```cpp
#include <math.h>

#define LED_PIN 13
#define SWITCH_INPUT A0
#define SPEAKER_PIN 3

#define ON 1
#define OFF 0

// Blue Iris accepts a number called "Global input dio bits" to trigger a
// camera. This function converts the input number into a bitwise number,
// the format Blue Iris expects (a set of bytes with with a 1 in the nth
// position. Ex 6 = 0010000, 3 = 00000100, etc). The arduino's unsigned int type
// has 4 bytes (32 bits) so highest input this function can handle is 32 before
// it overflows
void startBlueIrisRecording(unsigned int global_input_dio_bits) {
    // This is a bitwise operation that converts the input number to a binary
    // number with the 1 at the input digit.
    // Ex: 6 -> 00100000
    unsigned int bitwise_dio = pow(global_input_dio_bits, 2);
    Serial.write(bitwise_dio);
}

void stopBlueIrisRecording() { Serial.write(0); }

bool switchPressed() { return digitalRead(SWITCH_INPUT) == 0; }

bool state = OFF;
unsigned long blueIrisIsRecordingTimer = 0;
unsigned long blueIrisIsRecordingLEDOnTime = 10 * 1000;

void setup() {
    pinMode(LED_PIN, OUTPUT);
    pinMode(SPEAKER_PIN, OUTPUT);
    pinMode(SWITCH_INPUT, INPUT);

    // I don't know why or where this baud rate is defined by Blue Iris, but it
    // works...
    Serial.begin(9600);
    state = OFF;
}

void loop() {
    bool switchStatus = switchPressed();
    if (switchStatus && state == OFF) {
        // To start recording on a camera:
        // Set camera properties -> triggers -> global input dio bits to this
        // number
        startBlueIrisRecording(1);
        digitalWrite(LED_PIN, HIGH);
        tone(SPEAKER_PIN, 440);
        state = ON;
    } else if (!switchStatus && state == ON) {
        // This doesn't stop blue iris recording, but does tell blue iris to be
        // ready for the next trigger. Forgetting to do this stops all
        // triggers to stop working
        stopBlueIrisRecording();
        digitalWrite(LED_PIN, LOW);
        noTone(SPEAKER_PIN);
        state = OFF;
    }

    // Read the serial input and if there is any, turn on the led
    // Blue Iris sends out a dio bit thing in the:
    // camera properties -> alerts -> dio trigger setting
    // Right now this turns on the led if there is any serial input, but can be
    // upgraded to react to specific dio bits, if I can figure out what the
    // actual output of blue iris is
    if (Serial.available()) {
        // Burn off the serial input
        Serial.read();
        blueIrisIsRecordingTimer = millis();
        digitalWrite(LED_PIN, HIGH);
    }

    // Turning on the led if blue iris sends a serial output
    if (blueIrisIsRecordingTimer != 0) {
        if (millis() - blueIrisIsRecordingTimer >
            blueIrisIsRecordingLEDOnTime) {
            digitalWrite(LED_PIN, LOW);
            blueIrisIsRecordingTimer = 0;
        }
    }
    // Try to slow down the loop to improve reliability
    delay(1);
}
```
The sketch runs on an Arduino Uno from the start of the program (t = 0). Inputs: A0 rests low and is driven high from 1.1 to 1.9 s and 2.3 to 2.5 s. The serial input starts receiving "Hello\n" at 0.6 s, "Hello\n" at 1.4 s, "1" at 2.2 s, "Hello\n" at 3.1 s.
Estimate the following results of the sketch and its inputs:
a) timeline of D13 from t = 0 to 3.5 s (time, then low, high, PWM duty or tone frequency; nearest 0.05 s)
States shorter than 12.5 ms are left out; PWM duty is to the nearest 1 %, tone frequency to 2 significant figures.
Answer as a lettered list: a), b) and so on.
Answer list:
a) 0 s high; 1.1 s low; 1.4 s high; 2.3 s low; 2.5 s high
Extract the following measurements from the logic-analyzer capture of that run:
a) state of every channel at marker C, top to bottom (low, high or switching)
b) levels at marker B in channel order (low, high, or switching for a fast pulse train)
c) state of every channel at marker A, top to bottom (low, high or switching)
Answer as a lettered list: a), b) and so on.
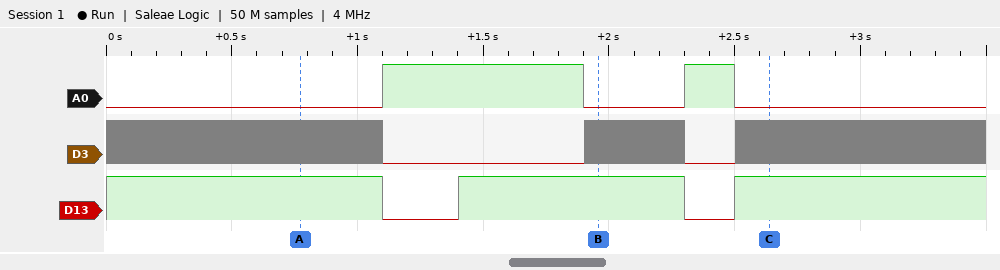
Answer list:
a) A0 low, D3 switching, D13 high
b) A0 low, D3 switching, D13 high
c) A0 low, D3 switching, D13 high
